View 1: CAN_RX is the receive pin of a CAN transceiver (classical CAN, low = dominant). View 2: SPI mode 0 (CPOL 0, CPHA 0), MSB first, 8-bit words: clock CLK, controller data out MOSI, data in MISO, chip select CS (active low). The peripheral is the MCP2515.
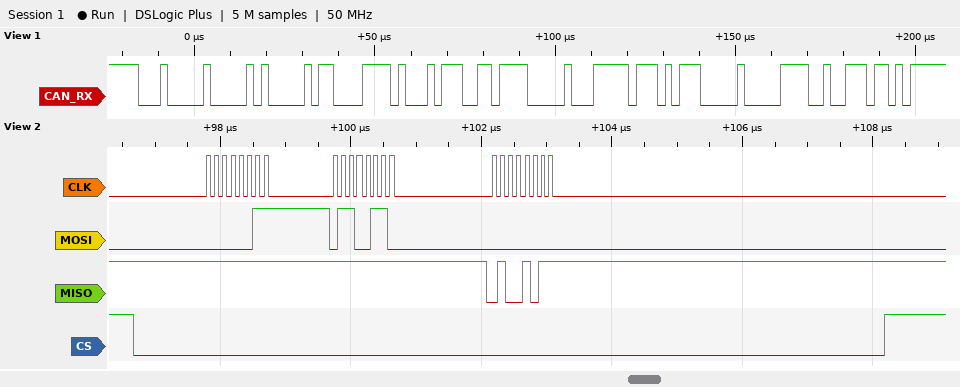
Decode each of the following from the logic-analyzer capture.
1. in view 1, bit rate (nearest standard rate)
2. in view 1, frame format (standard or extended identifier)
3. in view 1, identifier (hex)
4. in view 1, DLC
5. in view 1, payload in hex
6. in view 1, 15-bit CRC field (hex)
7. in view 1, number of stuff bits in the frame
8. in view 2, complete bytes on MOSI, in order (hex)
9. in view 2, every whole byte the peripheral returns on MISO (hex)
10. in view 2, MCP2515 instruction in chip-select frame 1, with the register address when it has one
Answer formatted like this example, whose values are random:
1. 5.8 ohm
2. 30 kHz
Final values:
1. 500 kbit/s
2. standard
3. 0x100
4. 8
5. 18 7A 2E 6F 00 FF 5C 00
6. 0x7276
7. 7
8. 03 66 00
9. FF FF 4B
10. READ 0x66
